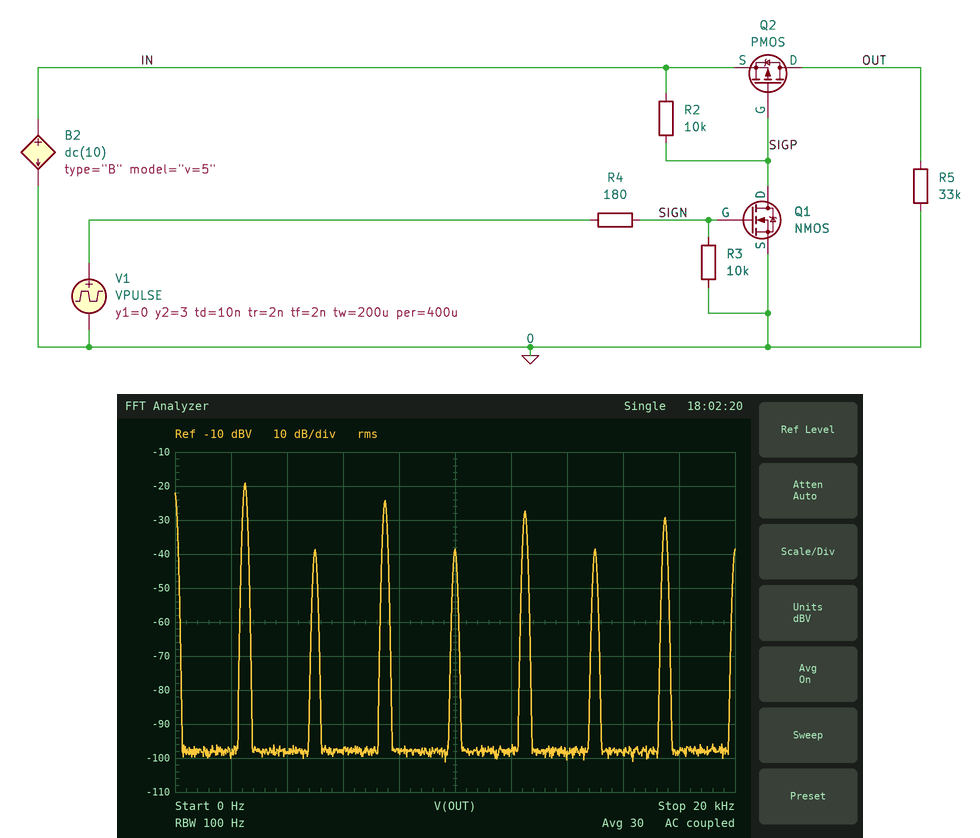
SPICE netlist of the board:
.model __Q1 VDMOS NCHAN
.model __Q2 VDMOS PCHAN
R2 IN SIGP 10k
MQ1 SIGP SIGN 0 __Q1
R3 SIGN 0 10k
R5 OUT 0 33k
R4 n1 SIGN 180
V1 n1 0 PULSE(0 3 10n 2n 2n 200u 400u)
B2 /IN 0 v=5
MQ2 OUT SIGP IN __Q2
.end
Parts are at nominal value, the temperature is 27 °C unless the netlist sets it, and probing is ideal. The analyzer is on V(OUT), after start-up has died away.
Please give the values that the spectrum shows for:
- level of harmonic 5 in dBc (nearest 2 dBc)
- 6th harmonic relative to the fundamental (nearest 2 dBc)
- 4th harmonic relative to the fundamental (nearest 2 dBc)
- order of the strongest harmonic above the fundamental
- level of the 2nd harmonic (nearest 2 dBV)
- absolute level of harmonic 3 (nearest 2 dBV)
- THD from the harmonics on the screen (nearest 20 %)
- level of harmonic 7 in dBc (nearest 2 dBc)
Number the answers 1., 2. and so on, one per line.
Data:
1. -8 dBc
2. -20 dBc
3. -20 dBc
4. 3
5. -38 dBV
6. -24 dBV
7. 80 %
8. -10 dBc
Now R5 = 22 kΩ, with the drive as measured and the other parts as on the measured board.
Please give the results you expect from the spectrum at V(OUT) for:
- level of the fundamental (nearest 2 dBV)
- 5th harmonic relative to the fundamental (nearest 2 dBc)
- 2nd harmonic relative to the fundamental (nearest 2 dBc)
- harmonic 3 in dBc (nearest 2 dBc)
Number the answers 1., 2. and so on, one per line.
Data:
1. -22 dBV
2. -6 dBc
3. -22 dBc
4. -4 dBc
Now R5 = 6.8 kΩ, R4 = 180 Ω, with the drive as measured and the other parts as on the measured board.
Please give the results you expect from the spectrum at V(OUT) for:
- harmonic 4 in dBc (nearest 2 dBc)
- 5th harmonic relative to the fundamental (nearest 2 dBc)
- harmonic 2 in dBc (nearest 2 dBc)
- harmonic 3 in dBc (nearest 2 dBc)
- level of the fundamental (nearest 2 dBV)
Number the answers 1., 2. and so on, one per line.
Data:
1. -18 dBc
2. -2 dBc
3. -24 dBc
4. 0 dBc
5. -30 dBV
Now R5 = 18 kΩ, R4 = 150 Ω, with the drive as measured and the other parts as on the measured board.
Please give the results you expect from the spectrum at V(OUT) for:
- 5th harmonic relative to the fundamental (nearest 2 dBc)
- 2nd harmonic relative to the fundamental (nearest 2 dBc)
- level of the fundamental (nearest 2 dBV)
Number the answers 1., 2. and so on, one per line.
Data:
1. -6 dBc
2. -24 dBc
3. -22 dBV
